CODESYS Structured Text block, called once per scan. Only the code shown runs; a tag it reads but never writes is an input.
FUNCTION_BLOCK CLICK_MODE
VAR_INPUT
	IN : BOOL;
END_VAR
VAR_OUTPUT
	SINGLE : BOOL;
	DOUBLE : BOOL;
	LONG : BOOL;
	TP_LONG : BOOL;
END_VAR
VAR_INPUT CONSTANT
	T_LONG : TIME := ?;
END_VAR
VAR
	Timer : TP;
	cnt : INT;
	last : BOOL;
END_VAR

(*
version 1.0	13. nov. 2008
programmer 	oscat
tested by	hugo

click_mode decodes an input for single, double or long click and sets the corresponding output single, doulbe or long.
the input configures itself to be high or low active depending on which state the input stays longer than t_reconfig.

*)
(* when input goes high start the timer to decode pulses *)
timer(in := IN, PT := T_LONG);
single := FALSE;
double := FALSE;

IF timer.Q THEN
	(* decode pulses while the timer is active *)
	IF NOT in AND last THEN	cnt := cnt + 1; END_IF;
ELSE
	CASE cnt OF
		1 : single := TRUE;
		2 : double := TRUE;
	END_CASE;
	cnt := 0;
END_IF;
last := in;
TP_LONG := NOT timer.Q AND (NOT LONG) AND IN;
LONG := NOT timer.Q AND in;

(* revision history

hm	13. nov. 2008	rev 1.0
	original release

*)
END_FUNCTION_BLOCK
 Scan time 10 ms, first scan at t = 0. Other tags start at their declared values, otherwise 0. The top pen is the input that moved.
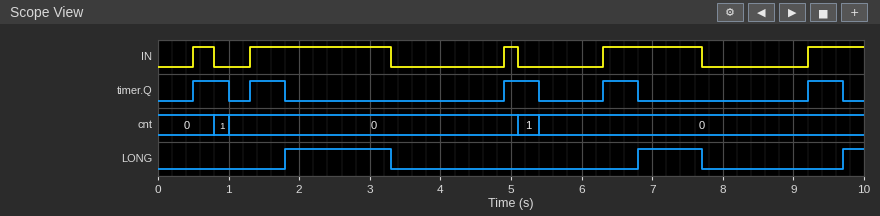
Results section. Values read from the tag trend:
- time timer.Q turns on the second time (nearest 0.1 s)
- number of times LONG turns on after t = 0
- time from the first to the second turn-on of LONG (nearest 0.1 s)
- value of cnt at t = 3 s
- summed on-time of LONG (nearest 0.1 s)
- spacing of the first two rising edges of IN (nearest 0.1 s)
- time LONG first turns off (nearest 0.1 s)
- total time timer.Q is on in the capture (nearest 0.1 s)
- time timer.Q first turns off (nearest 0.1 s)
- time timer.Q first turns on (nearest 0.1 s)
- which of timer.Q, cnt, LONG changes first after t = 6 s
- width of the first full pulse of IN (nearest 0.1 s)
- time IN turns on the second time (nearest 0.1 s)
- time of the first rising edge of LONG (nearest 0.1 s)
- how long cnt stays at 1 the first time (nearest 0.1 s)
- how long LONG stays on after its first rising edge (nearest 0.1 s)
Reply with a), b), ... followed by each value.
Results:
a) 1.3 s
b) 3
c) 5.0 s
d) 0
e) 2.7 s
f) 0.8 s
g) 3.3 s
h) 2.5 s
i) 1.0 s
j) 0.5 s
k) timer.Q
l) 0.3 s
m) 1.3 s
n) 1.8 s
o) 0.2 s
p) 1.5 s
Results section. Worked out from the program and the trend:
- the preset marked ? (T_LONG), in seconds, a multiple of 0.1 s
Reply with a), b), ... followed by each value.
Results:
a) 0.5 s
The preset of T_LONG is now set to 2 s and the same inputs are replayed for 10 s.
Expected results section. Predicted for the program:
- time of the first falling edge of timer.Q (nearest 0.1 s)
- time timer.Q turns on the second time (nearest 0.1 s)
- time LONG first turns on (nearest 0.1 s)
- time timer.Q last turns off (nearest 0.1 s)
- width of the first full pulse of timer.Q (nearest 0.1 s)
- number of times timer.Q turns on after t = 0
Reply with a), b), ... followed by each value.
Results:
a) 2.5 s
b) 4.9 s
c) 2.5 s
d) 6.9 s
e) 2.0 s
f) 3
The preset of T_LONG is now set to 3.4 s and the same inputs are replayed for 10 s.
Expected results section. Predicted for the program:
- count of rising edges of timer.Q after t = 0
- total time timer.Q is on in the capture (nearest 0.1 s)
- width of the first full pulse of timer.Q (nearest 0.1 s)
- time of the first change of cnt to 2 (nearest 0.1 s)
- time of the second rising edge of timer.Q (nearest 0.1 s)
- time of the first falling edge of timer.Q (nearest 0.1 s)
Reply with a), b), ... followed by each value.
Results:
a) 3
b) 7.6 s
c) 3.4 s
d) 3.3 s
e) 4.9 s
f) 3.9 s
